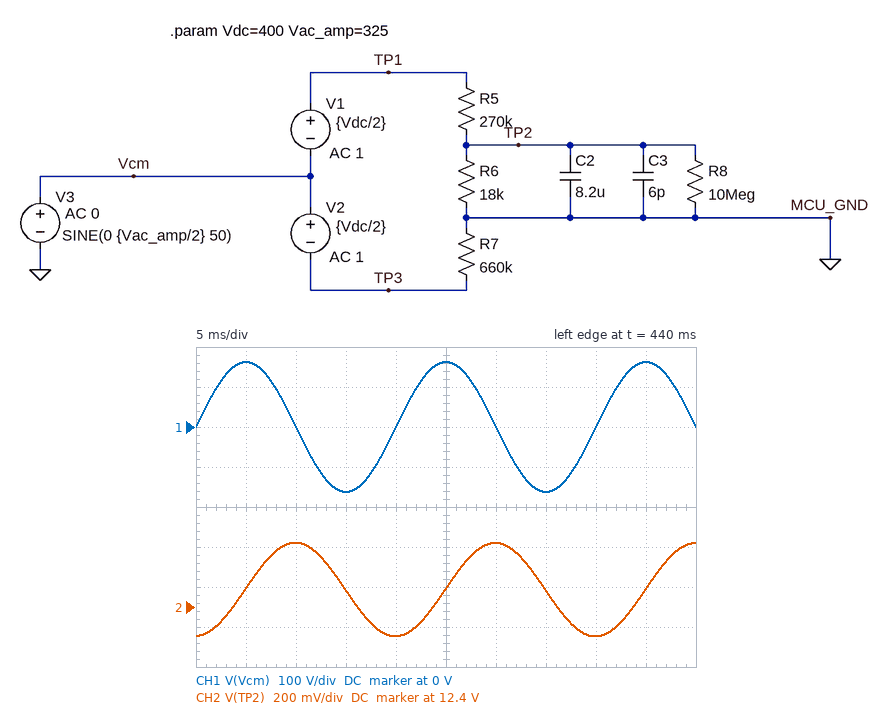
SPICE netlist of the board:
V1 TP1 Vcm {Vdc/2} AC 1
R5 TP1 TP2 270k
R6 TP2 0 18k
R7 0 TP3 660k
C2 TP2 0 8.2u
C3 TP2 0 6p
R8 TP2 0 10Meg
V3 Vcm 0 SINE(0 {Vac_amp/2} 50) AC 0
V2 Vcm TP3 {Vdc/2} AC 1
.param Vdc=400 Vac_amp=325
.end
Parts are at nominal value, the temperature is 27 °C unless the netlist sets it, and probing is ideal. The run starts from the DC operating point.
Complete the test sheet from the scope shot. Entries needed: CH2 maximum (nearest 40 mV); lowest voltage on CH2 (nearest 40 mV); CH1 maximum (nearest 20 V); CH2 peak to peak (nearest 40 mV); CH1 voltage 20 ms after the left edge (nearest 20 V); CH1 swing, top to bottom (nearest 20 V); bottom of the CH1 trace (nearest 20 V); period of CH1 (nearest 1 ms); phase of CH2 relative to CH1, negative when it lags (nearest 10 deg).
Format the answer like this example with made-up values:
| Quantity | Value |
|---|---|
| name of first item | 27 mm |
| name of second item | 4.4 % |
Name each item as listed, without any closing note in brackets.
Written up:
| Quantity | Value |
|---|---|
| CH2 maximum | 12.72 V |
| lowest voltage on CH2 | 12.24 V |
| CH1 maximum | 160 V |
| CH2 peak to peak | 480 mV |
| CH1 voltage 20 ms after the left edge | 0 V |
| CH1 swing, top to bottom | 320 V |
| bottom of the CH1 trace | -160 V |
| period of CH1 | 20 ms |
| phase of CH2 relative to CH1, negative when it lags | -90 deg |
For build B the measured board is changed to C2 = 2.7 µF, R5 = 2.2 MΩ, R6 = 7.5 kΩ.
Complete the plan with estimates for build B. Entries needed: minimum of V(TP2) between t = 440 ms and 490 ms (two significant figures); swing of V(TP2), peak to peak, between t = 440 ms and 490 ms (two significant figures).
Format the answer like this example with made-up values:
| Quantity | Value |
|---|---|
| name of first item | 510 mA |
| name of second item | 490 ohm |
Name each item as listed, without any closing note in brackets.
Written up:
| Quantity | Value |
|---|---|
| minimum of V(TP2) between t = 440 ms and 490 ms | 590 mV |
| swing of V(TP2), peak to peak, between t = 440 ms and 490 ms | 170 mV |
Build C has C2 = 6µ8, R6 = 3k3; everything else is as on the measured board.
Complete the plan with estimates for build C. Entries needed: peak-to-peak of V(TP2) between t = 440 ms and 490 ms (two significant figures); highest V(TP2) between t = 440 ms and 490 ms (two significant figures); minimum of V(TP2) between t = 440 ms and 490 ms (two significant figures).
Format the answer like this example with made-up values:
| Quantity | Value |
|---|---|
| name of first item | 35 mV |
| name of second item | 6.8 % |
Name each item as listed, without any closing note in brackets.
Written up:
| Quantity | Value |
|---|---|
| peak-to-peak of V(TP2) between t = 440 ms and 490 ms | 560 mV |
| highest V(TP2) between t = 440 ms and 490 ms | 2.7 V |
| minimum of V(TP2) between t = 440 ms and 490 ms | 2.1 V |
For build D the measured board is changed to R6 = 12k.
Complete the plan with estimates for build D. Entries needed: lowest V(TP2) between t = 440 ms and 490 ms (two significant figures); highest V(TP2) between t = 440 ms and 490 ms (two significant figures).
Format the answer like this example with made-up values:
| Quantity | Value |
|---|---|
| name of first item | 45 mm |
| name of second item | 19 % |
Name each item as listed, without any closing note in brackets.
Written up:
| Quantity | Value |
|---|---|
| lowest V(TP2) between t = 440 ms and 490 ms | 8.3 V |
| highest V(TP2) between t = 440 ms and 490 ms | 8.7 V |
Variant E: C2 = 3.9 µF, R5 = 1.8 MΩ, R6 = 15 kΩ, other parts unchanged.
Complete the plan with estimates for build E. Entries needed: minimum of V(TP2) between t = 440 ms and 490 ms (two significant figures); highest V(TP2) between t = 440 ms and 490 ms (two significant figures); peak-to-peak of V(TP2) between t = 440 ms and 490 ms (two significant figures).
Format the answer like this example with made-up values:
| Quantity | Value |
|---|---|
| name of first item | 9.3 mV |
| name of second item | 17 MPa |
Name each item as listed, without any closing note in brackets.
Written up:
| Quantity | Value |
|---|---|
| minimum of V(TP2) between t = 440 ms and 490 ms | 1.6 V |
| highest V(TP2) between t = 440 ms and 490 ms | 1.7 V |
| peak-to-peak of V(TP2) between t = 440 ms and 490 ms | 150 mV |
